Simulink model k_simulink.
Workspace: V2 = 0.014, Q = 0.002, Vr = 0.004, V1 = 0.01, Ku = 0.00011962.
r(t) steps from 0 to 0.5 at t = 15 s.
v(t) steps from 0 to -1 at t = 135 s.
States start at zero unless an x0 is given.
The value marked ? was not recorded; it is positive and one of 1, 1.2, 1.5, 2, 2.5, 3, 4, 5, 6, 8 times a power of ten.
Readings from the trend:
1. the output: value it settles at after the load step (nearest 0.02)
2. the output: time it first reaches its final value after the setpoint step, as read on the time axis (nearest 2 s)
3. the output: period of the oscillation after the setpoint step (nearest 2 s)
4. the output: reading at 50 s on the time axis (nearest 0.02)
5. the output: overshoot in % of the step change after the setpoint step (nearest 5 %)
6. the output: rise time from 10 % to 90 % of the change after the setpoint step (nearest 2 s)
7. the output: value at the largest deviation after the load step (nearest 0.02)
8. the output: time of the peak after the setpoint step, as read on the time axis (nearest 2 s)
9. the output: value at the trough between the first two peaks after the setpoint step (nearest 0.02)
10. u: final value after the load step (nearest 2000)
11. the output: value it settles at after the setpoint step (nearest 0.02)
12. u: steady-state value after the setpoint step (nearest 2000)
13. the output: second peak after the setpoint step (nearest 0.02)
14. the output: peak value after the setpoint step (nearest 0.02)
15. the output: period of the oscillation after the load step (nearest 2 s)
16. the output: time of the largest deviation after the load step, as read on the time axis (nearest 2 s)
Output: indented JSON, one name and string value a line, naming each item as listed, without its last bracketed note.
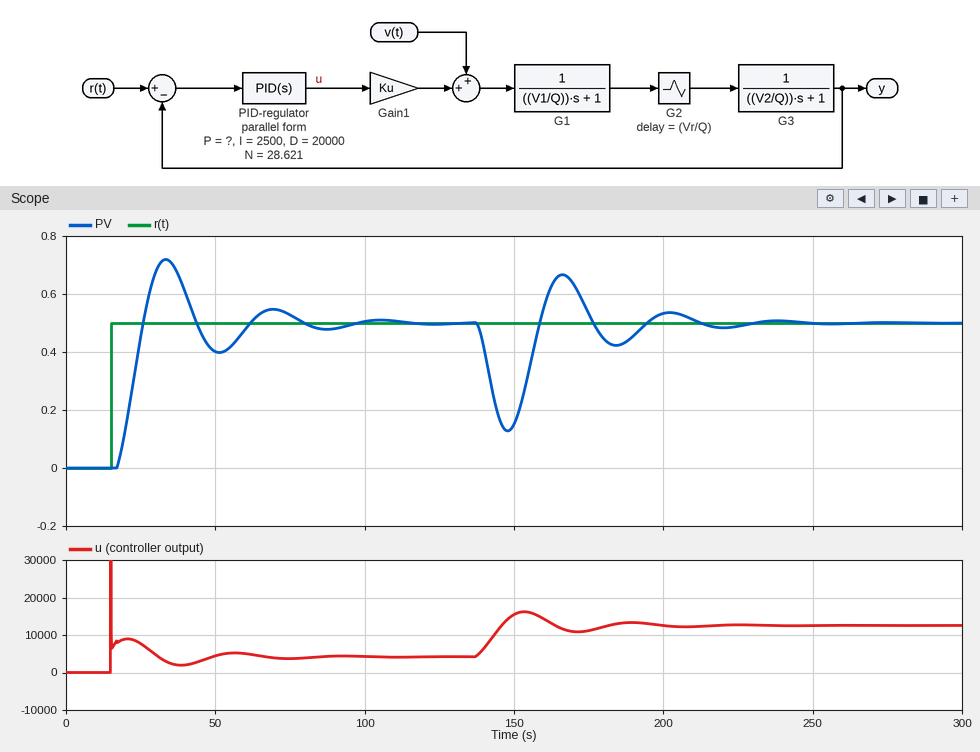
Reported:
{
  "the output: value it settles at after the load step": "0.50",
  "the output: time it first reaches its final value after the setpoint step, as read on the time axis": "26 s",
  "the output: period of the oscillation after the setpoint step": "36 s",
  "the output: reading at 50 s on the time axis": "0.40",
  "the output: overshoot in % of the step change after the setpoint step": "45 %",
  "the output: rise time from 10 % to 90 % of the change after the setpoint step": "6 s",
  "the output: value at the largest deviation after the load step": "0.12",
  "the output: time of the peak after the setpoint step, as read on the time axis": "34 s",
  "the output: value at the trough between the first two peaks after the setpoint step": "0.40",
  "u: final value after the load step": "12000",
  "the output: value it settles at after the setpoint step": "0.50",
  "u: steady-state value after the setpoint step": "4000",
  "the output: second peak after the setpoint step": "0.54",
  "the output: peak value after the setpoint step": "0.72",
  "the output: period of the oscillation after the load step": "36 s",
  "the output: time of the largest deviation after the load step, as read on the time axis": "148 s"
}
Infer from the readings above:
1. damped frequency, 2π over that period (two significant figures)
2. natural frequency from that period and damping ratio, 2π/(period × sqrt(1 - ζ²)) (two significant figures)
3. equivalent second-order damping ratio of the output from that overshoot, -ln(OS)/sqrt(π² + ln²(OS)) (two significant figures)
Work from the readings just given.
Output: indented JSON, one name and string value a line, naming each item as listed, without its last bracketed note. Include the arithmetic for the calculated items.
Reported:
{
  "damped frequency, 2π over that period": "2π / 36 = 0.17 rad/s",
  "natural frequency from that period and damping ratio, 2π/(period × sqrt(1 - ζ²))": "2π / (36 × sqrt(1 - 0.25²)) = 0.18 rad/s",
  "equivalent second-order damping ratio of the output from that overshoot, -ln(OS)/sqrt(π² + ln²(OS))": "ln(0.45) = -0.799; 0.799 / sqrt(9.870 + 0.638) = 0.25"
}
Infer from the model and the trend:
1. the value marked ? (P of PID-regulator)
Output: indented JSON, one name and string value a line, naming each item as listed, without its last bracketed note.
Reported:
{
  "the value marked ?": "12000"
}
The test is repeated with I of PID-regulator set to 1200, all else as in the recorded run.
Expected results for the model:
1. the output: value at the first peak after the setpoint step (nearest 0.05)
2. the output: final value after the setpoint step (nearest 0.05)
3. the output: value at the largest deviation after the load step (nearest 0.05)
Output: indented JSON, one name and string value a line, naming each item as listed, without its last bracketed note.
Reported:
{
  "the output: value at the first peak after the setpoint step": "0.55",
  "the output: final value after the setpoint step": "0.50",
  "the output: value at the largest deviation after the load step": "0.10"
}
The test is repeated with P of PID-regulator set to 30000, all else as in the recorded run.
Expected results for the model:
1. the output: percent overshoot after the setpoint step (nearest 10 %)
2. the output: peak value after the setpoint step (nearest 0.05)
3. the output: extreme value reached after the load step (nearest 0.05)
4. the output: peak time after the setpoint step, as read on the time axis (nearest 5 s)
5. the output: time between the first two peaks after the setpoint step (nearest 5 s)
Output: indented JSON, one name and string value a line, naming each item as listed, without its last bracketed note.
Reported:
{
  "the output: percent overshoot after the setpoint step": "50 %",
  "the output: peak value after the setpoint step": "0.75",
  "the output: extreme value reached after the load step": "0.20",
  "the output: peak time after the setpoint step, as read on the time axis": "25 s",
  "the output: time between the first two peaks after the setpoint step": "20 s"
}
